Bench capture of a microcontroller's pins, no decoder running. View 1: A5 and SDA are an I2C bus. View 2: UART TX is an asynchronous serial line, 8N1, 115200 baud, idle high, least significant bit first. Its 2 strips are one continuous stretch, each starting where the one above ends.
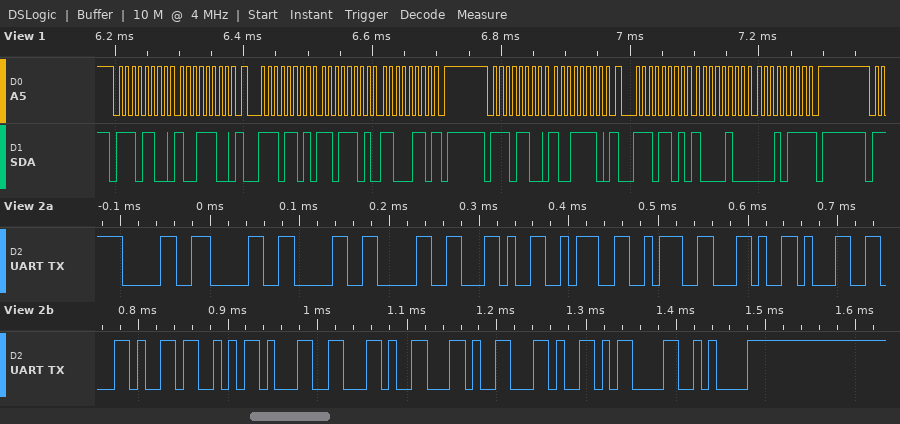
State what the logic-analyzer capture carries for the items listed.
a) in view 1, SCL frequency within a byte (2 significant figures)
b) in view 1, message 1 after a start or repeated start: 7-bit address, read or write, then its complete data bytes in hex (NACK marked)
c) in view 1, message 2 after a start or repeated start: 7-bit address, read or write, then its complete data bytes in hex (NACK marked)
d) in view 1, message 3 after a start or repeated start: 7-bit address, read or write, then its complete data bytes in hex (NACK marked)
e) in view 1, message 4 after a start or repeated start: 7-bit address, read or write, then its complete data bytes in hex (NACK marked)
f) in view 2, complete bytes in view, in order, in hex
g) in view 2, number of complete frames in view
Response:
100 kHz
0x76 write: 9C
0x76 read: DD C6 NACK
0x76 write: 9E
0x76 read: 84 17 NACK
0x30 0x30 0x30 0x30 0x2C 0x3A 0x3A 0x2C 0x31 0x2C 0x53 0x31 0x2C 0x2C 0x2C 0x0D 0x0A
17
